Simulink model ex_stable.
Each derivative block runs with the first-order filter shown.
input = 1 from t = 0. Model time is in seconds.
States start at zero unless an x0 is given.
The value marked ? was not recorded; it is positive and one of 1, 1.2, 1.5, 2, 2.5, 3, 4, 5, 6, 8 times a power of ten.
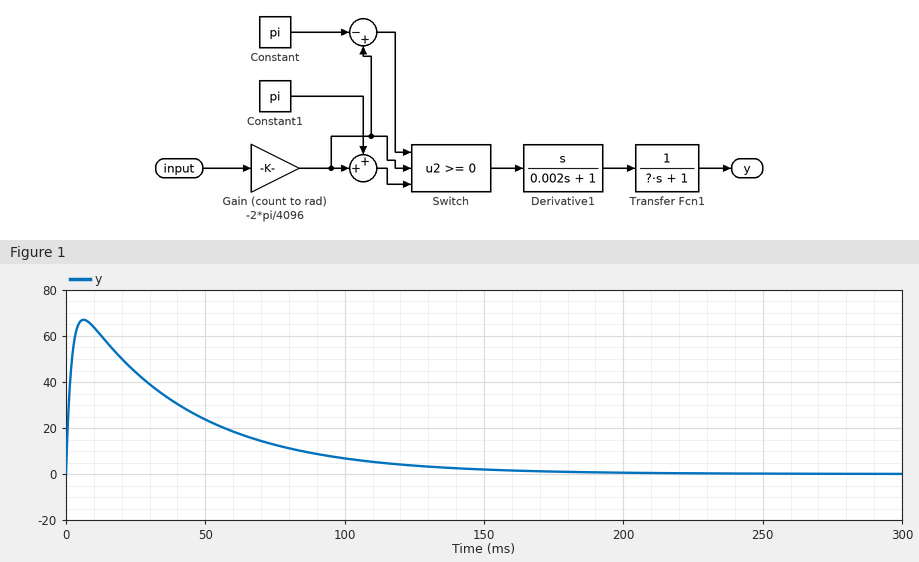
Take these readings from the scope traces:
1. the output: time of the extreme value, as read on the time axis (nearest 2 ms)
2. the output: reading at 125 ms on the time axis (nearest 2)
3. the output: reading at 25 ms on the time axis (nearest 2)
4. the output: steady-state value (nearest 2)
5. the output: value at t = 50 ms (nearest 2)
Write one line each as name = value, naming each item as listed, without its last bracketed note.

the output: time of the extreme value, as read on the time axis = 6 ms
the output: reading at 125 ms on the time axis = 4
the output: reading at 25 ms on the time axis = 44
the output: steady-state value = 0
the output: value at t = 50 ms = 24
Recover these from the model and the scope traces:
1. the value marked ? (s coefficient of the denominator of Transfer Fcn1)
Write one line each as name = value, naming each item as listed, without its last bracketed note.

the value marked ? = 0.04
